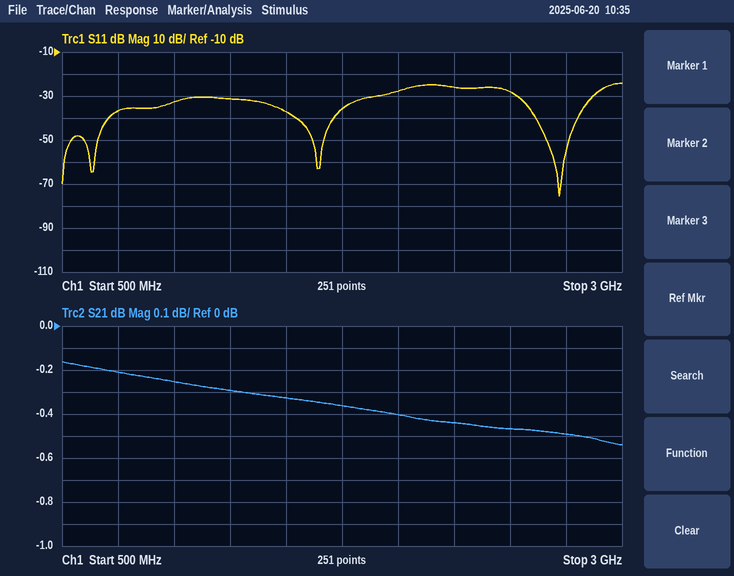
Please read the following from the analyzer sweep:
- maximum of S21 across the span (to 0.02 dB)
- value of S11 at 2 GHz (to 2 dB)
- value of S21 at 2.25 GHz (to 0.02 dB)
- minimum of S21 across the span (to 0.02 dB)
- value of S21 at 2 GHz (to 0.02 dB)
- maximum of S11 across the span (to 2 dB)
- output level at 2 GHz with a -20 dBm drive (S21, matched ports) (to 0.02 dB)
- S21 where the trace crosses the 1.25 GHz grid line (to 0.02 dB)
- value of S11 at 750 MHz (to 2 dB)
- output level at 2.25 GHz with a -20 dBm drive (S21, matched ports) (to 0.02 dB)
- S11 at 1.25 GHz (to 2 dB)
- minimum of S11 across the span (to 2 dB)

-0.16 dB
-28 dB
-0.44 dB
-0.54 dB
-0.40 dB
-24 dB
-20.40 dBm
-0.30 dB
-36 dB
-20.44 dBm
-32 dB
-76 dB
